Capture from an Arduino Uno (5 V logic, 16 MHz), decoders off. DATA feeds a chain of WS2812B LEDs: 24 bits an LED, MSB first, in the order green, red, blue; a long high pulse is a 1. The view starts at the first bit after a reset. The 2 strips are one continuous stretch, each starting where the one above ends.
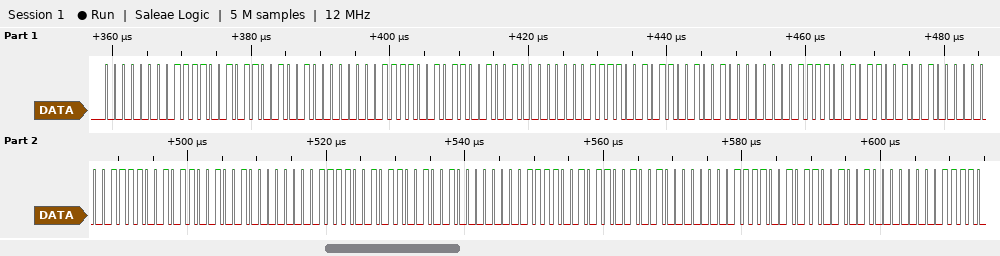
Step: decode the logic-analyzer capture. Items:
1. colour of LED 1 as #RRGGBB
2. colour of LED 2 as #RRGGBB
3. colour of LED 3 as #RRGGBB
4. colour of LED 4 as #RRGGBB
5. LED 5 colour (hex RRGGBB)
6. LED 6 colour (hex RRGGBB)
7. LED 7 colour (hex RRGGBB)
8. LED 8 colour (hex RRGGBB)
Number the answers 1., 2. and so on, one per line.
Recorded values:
1. #F200C9
2. #F200C9
3. #F200C9
4. #F200C9
5. #F200C9
6. #F200C9
7. #F200C9
8. #F200C9
